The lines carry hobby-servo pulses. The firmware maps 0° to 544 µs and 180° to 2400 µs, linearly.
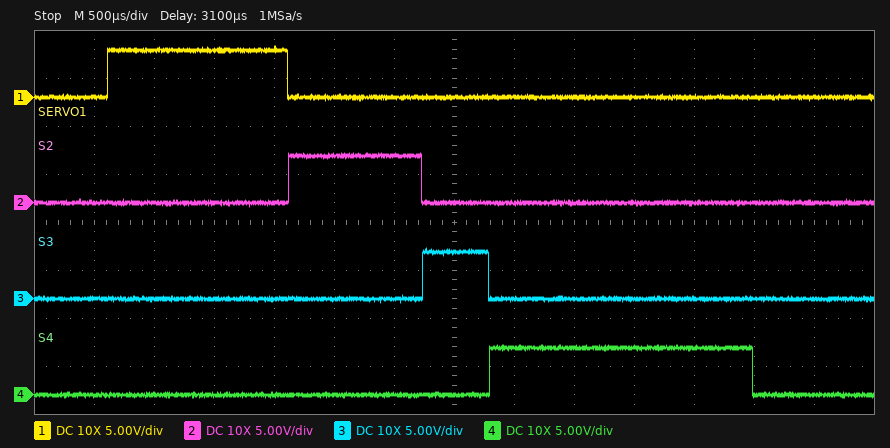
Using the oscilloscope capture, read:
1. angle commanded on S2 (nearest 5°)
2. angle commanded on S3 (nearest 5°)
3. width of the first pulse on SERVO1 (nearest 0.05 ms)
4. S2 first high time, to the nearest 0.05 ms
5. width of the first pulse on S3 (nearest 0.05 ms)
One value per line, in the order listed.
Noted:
55°
0°
1.50 ms
1.10 ms
0.55 ms
